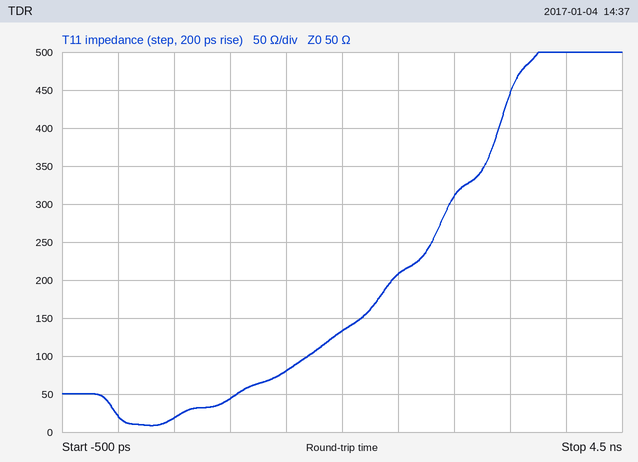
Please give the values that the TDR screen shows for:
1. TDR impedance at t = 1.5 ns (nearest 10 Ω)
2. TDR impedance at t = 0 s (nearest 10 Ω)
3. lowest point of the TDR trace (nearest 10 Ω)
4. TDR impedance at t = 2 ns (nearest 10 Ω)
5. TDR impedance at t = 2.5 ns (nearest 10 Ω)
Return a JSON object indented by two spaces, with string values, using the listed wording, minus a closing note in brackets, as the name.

{
  "TDR impedance at t = 1.5 ns": "80 Ω",
  "TDR impedance at t = 0 s": "20 Ω",
  "lowest point of the TDR trace": "10 Ω",
  "TDR impedance at t = 2 ns": "130 Ω",
  "TDR impedance at t = 2.5 ns": "210 Ω"
}
